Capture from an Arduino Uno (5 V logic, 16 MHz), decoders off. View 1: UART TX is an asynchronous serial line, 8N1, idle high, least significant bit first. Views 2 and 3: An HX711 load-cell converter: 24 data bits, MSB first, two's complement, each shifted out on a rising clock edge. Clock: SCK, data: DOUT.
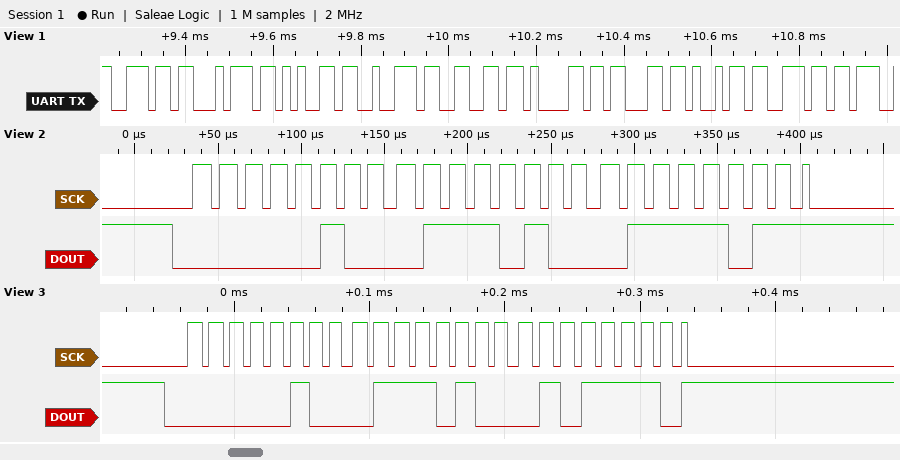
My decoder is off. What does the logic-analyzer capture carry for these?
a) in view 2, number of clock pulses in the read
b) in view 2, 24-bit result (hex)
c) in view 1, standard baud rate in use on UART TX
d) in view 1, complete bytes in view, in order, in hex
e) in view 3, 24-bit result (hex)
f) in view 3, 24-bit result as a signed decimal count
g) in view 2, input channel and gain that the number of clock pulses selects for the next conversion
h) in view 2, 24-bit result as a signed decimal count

25
0x04747B
57600 baud
6E 74 65 72 66 61 63 69 6E
0x04745E
291934
channel A, gain 128
291963
